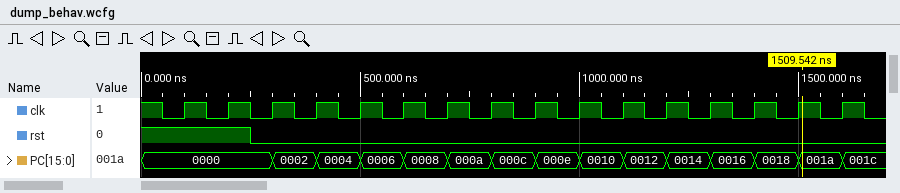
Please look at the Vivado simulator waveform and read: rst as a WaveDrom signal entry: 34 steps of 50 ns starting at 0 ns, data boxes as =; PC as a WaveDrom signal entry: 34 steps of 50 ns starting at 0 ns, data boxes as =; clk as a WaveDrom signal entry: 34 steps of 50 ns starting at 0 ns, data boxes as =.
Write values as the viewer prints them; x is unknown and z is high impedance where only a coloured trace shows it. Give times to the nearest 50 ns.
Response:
{name: 'rst', wave: '1....0............................'}
{name: 'PC', wave: '=.....=.=.=.=.=.=.=.=.=.=.=.=.=.=.', data: '0000 0002 0004 0006 0008 000a 000c 000e 0010 0012 0014 0016 0018 001a 001c'}
{name: 'clk', wave: '1010101010101010101010101010101010'}
